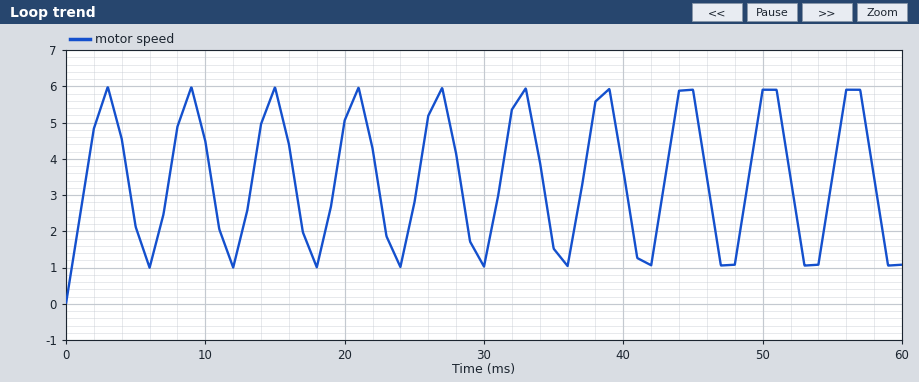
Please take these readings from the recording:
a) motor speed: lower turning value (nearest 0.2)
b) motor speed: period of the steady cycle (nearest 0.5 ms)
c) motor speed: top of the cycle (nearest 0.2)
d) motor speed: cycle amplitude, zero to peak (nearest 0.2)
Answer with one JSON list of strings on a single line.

["1.0", "6.0 ms", "6.0", "2.4"]
